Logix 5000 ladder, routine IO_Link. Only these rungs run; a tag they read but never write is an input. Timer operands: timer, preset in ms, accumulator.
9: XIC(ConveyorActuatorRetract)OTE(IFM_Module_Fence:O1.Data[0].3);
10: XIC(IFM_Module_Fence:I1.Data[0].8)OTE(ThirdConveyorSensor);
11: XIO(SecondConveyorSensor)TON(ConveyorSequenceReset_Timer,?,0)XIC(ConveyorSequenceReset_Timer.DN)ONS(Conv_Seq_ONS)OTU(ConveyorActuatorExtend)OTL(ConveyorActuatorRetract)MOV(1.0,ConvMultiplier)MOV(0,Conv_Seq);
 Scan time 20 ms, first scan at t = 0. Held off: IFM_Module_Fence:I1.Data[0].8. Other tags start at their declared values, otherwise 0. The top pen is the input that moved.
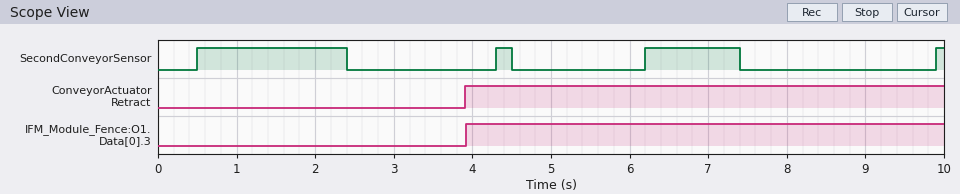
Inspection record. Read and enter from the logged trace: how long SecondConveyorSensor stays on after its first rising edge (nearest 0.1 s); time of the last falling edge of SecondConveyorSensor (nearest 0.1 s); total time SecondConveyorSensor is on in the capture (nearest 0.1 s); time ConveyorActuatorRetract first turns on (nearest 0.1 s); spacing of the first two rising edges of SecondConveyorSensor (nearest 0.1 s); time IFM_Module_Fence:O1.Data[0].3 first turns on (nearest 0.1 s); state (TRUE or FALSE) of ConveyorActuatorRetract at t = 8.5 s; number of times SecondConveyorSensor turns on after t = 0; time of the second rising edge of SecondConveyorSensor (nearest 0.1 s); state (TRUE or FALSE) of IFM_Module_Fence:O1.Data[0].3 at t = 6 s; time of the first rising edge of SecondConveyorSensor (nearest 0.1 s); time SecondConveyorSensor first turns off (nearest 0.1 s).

1.9 s
7.4 s
3.4 s
3.9 s
3.8 s
3.9 s
TRUE
4
4.3 s
TRUE
0.5 s
2.4 s
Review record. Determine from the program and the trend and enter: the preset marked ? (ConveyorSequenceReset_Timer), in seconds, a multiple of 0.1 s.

1.5 s
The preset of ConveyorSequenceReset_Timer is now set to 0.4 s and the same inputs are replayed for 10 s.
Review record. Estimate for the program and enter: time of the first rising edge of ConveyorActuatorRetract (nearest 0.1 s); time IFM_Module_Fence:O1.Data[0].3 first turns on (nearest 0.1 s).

0.4 s
0.4 s
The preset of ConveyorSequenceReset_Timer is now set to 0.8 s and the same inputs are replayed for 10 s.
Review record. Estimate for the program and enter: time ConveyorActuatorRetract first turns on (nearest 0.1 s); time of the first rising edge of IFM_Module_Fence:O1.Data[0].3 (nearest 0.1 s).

3.2 s
3.2 s
